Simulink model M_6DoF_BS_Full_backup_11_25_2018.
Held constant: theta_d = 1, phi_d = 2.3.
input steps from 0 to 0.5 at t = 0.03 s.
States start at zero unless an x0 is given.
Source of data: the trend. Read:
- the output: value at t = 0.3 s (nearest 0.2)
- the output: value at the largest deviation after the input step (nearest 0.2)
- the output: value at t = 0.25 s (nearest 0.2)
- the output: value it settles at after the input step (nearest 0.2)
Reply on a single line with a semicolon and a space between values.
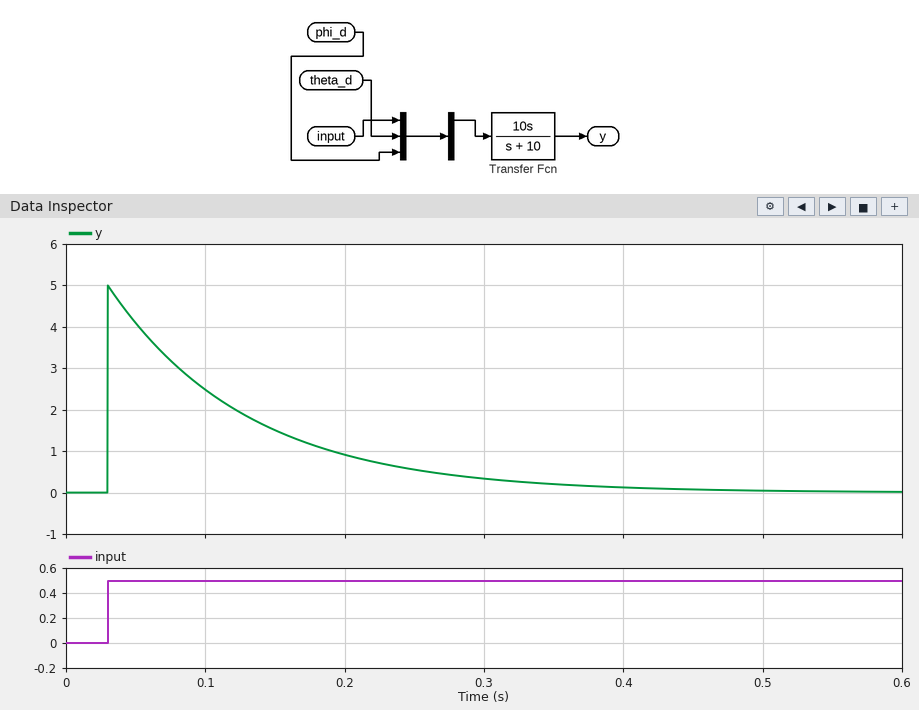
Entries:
0.4; 5.0; 0.6; 0.0
